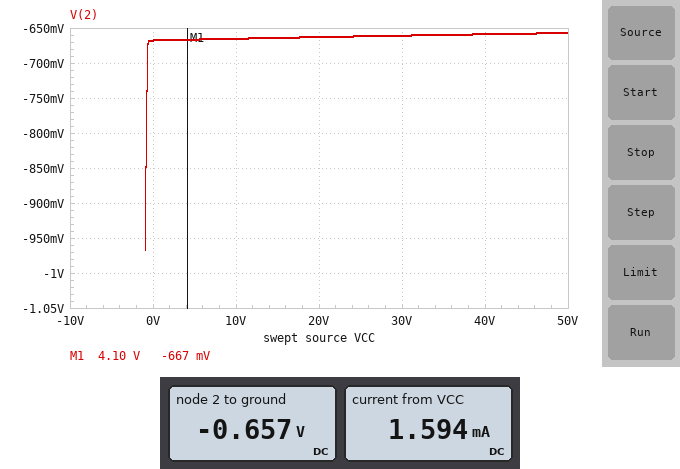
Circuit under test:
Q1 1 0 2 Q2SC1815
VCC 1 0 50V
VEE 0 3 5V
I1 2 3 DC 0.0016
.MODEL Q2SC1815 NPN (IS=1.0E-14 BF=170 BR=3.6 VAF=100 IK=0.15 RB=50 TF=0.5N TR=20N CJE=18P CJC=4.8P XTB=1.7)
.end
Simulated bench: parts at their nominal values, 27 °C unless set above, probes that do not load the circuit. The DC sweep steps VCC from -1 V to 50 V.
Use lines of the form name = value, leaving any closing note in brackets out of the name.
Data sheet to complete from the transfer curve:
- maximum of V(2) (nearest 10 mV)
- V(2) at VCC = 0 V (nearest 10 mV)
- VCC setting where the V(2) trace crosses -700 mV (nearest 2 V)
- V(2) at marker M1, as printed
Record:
maximum of V(2) = -660 mV
V(2) at VCC = 0 V = -670 mV
VCC setting where the V(2) trace crosses -700 mV = 0 V
V(2) at marker M1, as printed = -667 mV
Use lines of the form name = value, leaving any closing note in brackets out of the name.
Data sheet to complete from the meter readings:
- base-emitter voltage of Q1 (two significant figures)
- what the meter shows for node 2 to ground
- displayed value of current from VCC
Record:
base-emitter voltage of Q1 = 660 mV
what the meter shows for node 2 to ground = -0.657 V
displayed value of current from VCC = 1.594 mA
